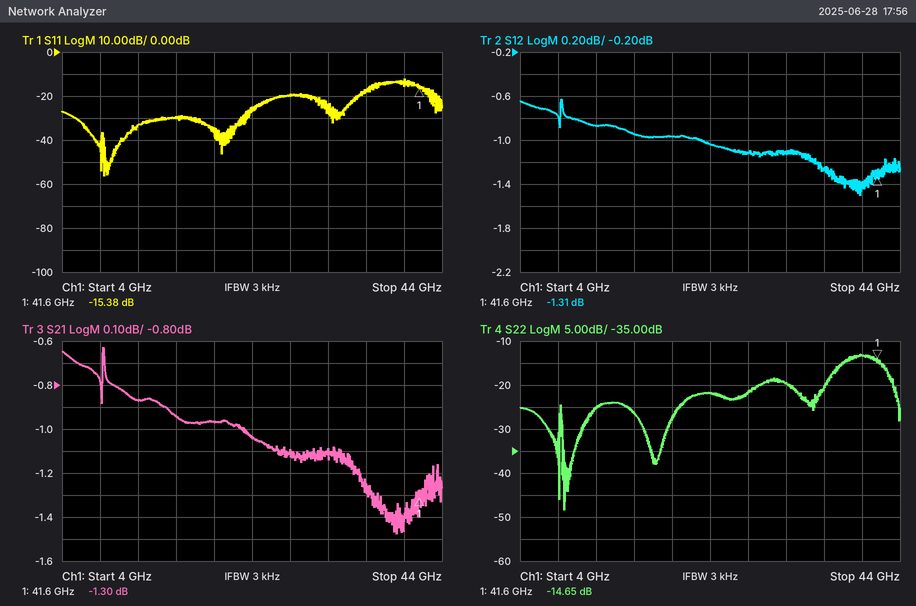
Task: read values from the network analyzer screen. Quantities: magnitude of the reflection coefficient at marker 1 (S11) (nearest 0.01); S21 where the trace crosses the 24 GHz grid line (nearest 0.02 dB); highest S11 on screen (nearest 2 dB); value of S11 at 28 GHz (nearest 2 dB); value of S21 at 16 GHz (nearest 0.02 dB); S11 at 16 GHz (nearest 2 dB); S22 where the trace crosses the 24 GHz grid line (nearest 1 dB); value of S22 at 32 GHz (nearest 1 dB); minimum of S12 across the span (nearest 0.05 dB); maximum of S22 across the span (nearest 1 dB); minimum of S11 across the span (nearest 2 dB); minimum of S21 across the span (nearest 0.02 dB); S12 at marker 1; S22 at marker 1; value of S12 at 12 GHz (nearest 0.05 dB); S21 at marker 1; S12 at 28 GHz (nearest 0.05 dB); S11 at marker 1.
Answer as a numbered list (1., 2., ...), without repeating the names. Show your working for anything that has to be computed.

1. 10^(-15.38/20) ≈ 0.17
2. -1.04 dB
3. -12 dB
4. -20 dB
5. -0.94 dB
6. -30 dB
7. -22 dB
8. -20 dB
9. -1.50 dB
10. -13 dB
11. -56 dB
12. -1.48 dB
13. -1.31 dB
14. -14.65 dB
15. -0.85 dB
16. -1.30 dB
17. -1.10 dB
18. -15.38 dB
